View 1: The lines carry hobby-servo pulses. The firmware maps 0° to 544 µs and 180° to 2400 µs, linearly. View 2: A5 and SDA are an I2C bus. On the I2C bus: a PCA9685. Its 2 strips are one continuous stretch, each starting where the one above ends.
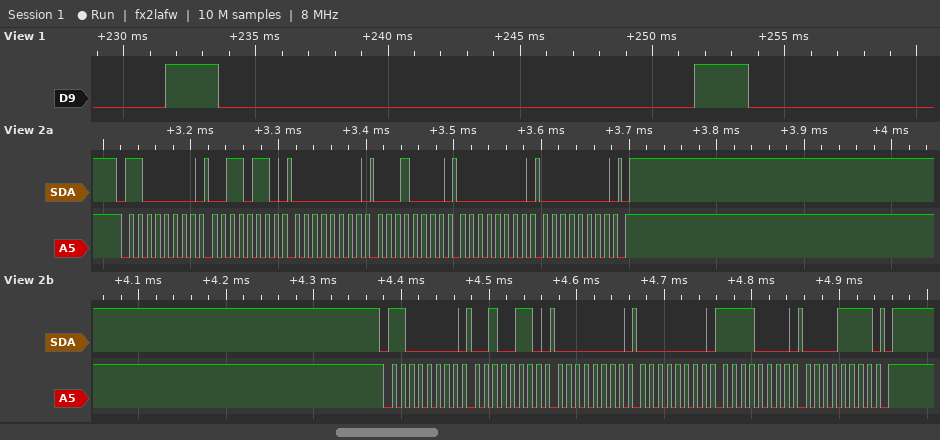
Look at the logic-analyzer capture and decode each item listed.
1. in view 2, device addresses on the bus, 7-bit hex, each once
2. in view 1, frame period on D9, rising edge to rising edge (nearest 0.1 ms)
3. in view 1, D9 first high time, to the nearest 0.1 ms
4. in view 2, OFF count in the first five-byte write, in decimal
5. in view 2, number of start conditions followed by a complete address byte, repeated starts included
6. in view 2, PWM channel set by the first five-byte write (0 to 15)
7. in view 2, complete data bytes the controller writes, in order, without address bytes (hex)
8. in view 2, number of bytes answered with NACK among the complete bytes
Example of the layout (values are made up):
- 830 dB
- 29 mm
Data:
- 0x60
- 20.0 ms
- 2.0 ms
- 0
- 2
- 12
- 36 00 10 00 00 26 00 00 F0 0F
- 0
